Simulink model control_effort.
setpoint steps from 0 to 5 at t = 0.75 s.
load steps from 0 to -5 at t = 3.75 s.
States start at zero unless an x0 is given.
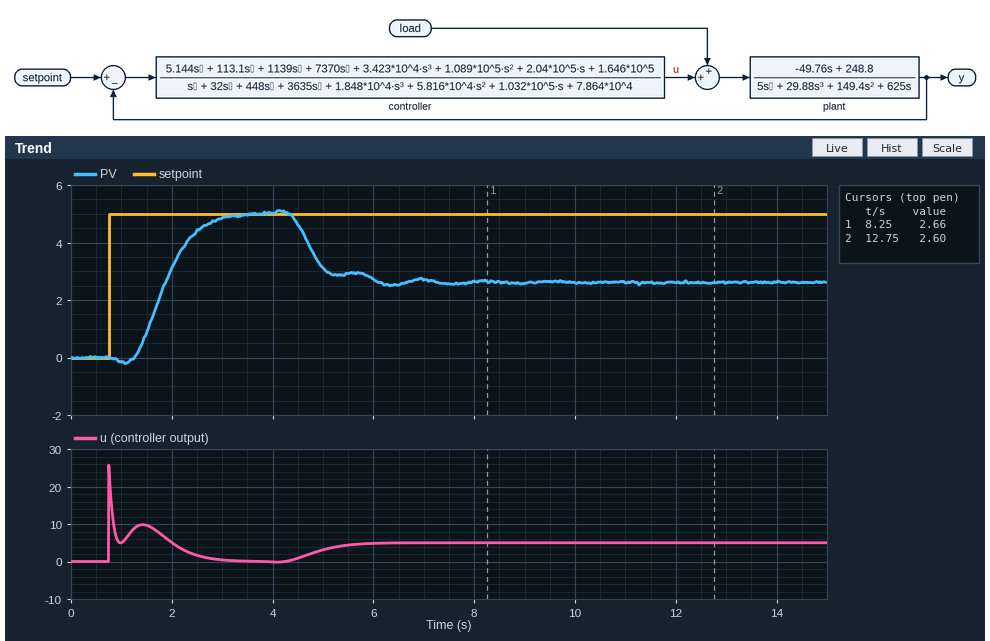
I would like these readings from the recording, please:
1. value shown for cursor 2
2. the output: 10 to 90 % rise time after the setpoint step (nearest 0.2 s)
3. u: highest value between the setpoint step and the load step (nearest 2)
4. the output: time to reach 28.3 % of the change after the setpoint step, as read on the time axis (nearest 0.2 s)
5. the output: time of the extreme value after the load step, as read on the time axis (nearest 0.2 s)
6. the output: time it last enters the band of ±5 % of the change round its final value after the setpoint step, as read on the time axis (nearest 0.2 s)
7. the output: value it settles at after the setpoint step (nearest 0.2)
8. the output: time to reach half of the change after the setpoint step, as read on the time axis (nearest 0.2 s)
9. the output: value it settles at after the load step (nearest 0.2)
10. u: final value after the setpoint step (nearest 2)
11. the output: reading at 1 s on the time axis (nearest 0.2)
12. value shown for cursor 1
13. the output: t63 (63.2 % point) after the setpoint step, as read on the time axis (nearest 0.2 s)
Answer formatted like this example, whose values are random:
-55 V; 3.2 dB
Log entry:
2.60; 1.2 s; 26; 1.6 s; 6.4 s; 2.8 s; 5.0; 1.8 s; 2.6; 0; -0.2; 2.66; 2.0 s
